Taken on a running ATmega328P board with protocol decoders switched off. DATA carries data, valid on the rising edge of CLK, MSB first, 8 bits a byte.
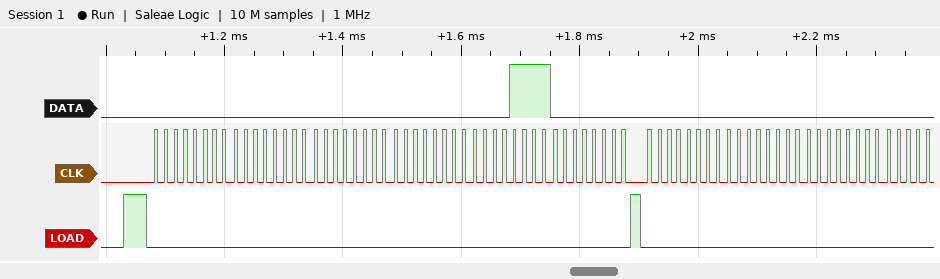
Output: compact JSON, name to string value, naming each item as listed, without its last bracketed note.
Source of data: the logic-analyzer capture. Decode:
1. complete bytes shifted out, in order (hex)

{"complete bytes shifted out, in order": "0x00 0x00 0x00 0x00 0x0F 0x00 0x00 0x00 0x00"}
